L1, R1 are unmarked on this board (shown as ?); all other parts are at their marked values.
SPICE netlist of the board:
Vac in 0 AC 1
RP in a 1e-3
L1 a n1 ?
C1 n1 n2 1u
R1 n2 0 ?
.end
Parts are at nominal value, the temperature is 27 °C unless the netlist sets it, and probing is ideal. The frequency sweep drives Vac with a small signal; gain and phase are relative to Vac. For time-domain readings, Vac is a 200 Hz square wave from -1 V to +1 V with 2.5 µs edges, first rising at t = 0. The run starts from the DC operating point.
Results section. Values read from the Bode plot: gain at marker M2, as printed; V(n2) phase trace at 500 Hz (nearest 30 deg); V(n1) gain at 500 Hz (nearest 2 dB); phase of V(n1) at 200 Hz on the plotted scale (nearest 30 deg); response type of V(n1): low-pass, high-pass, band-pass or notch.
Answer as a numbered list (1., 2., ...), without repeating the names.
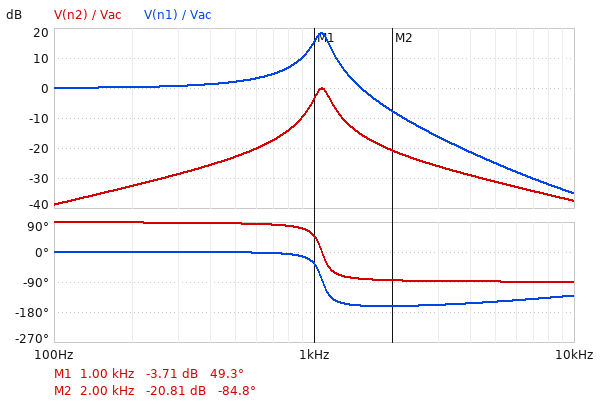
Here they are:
1. -20.81 dB
2. 90 deg
3. 2 dB
4. 0 deg
5. low-pass
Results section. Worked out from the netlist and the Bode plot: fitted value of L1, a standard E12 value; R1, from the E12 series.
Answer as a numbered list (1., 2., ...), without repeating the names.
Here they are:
1. 22 mH
2. 18 Ω
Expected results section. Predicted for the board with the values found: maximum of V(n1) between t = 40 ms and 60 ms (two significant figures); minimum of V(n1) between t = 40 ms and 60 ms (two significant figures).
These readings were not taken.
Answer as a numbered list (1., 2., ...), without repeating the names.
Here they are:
1. 2.9 V
2. -2.9 V
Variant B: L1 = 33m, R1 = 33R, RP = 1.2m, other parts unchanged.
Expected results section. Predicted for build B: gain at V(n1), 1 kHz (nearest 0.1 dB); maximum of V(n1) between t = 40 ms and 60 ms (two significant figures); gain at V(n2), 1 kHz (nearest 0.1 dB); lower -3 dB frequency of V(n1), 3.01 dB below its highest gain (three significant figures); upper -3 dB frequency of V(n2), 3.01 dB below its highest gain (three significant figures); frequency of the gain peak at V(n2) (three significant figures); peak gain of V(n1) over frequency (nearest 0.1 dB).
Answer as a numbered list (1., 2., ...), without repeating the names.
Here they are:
1. 8.9 dB
2. 2.3 V
3. -5.0 dB
4. 785 Hz
5. 959 Hz
6. 876 Hz
7. 15.0 dB
